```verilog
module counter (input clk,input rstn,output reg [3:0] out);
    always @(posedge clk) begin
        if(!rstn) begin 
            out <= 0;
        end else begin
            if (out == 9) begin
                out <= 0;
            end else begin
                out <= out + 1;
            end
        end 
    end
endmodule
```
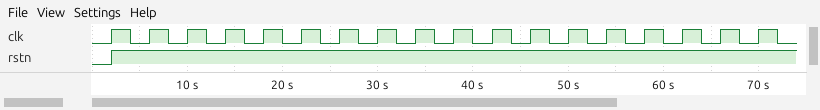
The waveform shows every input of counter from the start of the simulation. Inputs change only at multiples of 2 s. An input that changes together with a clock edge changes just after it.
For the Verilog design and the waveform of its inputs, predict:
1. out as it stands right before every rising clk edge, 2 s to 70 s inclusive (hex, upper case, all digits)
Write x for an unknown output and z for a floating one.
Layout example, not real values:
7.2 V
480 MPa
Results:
x, 0, 1, 2, 3, 4, 5, 6, 7, 8, 9, 0, 1, 2, 3, 4, 5, 6
